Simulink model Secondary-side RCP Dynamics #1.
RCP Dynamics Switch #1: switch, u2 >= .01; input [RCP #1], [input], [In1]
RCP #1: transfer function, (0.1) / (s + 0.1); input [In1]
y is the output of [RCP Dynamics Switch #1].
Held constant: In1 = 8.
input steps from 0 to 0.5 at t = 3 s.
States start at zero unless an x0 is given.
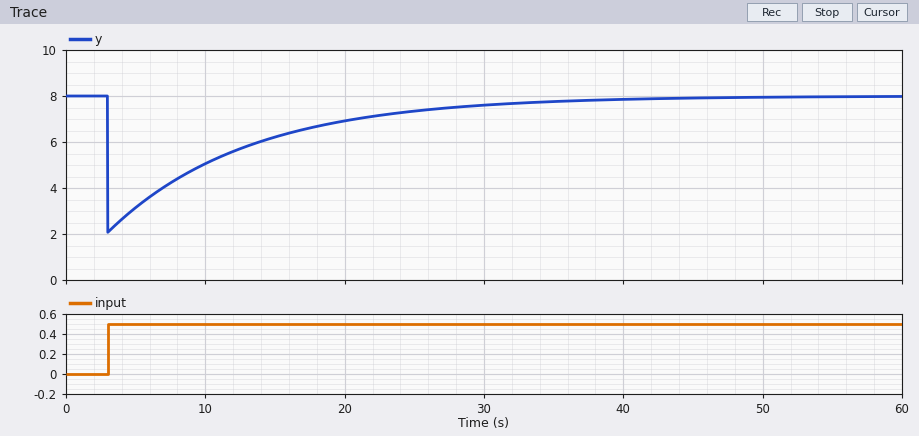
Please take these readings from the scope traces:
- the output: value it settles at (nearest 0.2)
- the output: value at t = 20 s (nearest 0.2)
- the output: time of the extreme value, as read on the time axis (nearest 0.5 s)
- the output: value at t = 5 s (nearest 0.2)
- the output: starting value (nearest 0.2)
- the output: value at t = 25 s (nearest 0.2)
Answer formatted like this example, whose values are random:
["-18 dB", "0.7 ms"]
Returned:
["8.0", "7.0", "3.0 s", "3.2", "8.0", "7.4"]
